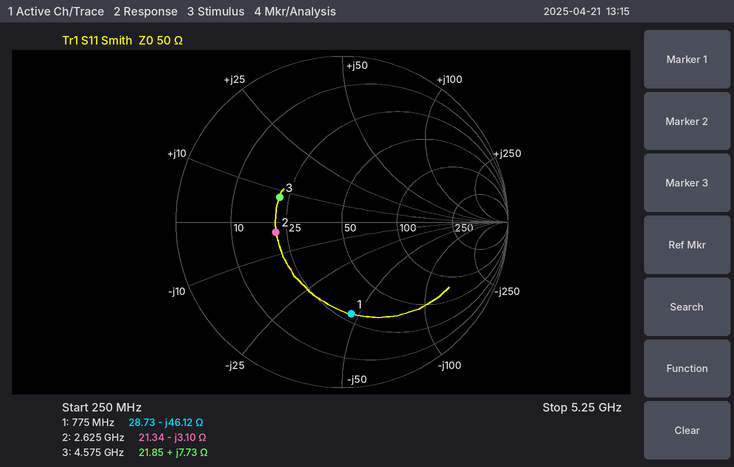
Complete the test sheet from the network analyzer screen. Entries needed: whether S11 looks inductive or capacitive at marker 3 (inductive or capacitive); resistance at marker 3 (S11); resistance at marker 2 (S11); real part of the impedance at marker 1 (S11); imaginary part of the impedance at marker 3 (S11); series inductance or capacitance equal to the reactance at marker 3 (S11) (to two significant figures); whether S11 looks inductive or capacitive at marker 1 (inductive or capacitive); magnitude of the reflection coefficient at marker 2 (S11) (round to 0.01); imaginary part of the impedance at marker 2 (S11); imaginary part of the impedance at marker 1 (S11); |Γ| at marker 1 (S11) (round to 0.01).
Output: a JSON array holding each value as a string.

["inductive", "21.85 Ω", "21.34 Ω", "28.73 Ω", "+7.73 Ω", "270 pH", "capacitive", "0.40", "-3.10 Ω", "-46.12 Ω", "0.56"]
